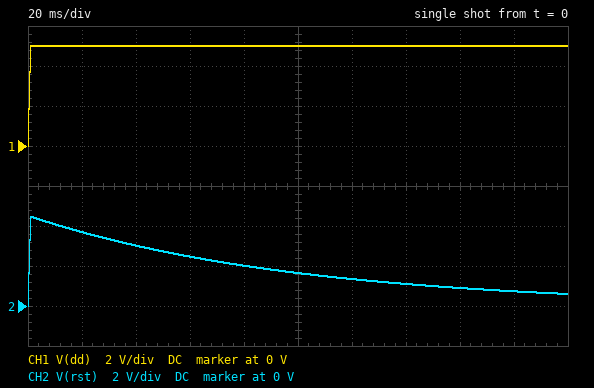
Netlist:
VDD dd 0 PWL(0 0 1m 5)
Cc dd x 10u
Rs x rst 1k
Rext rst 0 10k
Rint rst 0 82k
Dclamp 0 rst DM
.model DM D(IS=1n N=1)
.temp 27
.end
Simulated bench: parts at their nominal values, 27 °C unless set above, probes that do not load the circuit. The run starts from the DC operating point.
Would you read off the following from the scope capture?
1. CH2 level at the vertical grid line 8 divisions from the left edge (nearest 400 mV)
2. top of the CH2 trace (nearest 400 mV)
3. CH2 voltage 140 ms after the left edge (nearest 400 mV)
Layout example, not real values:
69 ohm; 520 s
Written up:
800 mV; 4.4 V; 1.2 V
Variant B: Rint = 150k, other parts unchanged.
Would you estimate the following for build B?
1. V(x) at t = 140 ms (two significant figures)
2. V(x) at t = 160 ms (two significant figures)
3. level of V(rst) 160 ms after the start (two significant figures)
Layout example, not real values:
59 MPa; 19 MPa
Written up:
1.3 V; 1.1 V; 970 mV
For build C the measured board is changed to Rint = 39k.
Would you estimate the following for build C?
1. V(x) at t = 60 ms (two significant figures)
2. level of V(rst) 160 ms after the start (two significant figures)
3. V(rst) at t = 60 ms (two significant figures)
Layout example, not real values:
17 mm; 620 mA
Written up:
2.6 V; 750 mV; 2.3 V
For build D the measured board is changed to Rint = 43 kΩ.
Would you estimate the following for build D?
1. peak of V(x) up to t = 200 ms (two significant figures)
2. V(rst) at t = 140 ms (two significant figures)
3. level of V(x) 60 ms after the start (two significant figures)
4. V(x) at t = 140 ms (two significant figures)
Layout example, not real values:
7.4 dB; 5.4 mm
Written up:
5.0 V; 960 mV; 2.6 V; 1.1 V
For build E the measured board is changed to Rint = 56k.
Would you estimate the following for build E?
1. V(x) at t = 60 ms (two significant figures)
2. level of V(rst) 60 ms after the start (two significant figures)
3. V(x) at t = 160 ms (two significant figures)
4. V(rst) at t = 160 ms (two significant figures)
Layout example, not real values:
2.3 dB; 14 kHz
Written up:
2.7 V; 2.4 V; 930 mV; 830 mV
